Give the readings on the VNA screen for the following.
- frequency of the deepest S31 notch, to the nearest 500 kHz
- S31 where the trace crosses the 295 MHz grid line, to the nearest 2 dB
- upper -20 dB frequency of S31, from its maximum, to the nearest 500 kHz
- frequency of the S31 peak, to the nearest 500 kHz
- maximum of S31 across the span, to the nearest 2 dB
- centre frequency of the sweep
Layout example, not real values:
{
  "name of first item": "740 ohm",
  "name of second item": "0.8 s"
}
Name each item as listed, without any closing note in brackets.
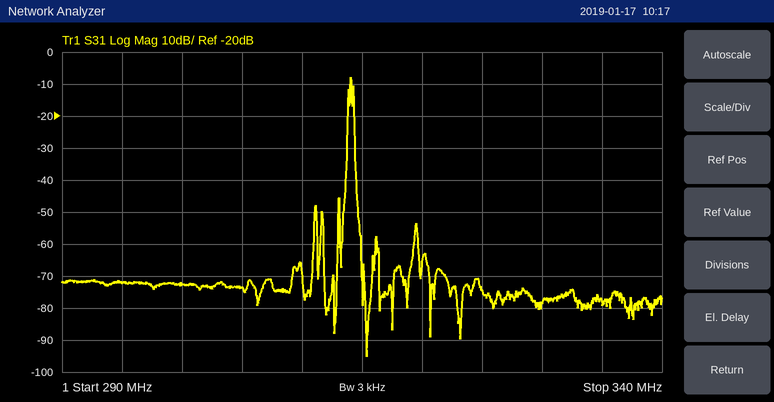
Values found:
{
  "frequency of the deepest S31 notch, to the nearest 500 kHz": "315.5 MHz",
  "S31 where the trace crosses the 295 MHz grid line, to the nearest 2 dB": "-72 dB",
  "upper -20 dB frequency of S31, from its maximum, to the nearest 500 kHz": "314.5 MHz",
  "frequency of the S31 peak, to the nearest 500 kHz": "314.0 MHz",
  "maximum of S31 across the span, to the nearest 2 dB": "-8 dB",
  "centre frequency of the sweep": "315 MHz"
}
